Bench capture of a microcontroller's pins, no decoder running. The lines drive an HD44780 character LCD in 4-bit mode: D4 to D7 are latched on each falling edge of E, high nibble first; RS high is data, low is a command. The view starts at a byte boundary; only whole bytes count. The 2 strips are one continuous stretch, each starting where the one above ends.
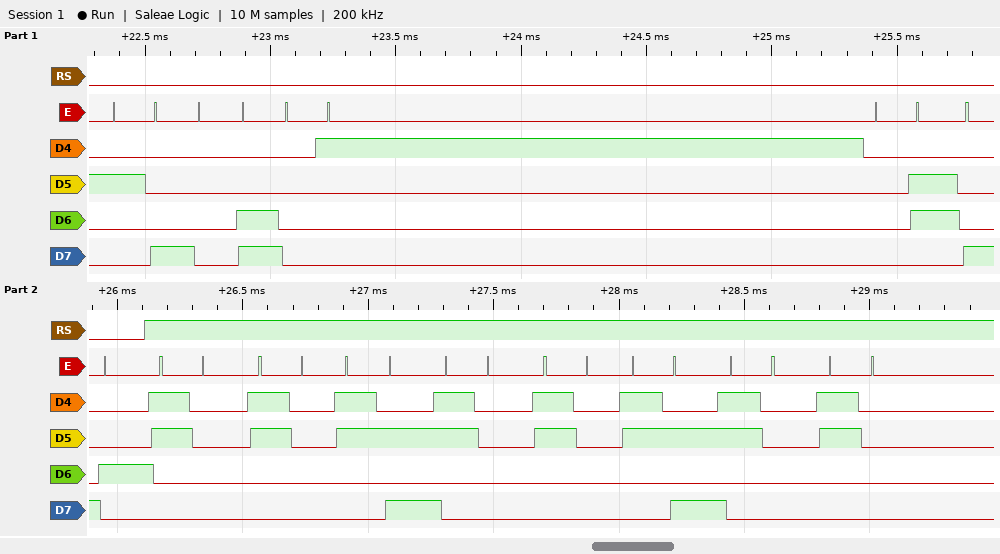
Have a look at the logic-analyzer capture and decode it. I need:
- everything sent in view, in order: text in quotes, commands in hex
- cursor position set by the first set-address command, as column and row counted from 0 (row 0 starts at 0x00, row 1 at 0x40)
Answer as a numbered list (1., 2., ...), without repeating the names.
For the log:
1. 0x28 0x0C 0x01 0x06 0x84 "00:00:00"
2. column 4, row 0
